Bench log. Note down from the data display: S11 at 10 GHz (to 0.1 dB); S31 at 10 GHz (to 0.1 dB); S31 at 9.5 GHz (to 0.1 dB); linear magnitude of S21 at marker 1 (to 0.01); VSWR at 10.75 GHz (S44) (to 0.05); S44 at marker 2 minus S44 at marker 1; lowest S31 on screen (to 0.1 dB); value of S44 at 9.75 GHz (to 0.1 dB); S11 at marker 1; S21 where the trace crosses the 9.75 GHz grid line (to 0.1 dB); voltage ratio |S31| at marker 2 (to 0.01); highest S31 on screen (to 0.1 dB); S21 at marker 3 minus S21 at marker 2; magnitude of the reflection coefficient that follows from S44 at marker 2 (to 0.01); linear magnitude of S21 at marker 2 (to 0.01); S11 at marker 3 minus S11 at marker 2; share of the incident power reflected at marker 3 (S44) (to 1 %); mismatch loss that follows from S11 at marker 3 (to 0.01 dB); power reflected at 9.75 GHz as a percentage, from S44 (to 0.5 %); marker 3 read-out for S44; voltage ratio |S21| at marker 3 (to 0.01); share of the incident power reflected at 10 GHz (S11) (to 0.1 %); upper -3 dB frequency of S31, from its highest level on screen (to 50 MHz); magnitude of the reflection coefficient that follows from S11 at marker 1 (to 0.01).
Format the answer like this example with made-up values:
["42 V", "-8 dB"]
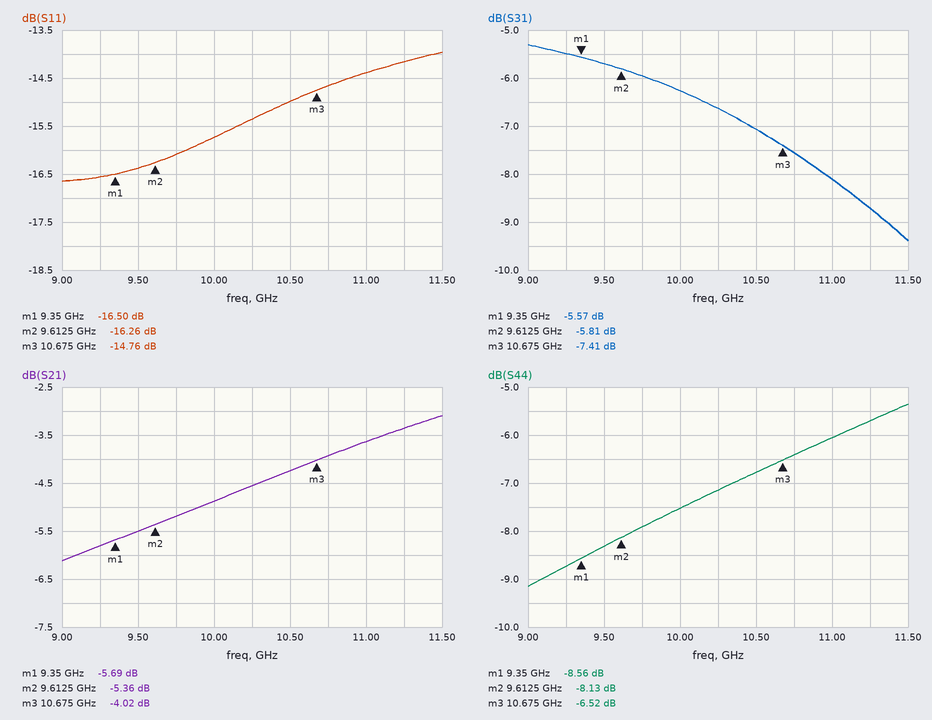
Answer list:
["-15.7 dB", "-6.3 dB", "-5.7 dB", "0.52", "2.85", "0.43 dB", "-9.4 dB", "-7.9 dB", "-16.50 dB", "-5.2 dB", "0.51", "-5.3 dB", "1.34 dB", "0.39", "0.54", "1.50 dB", "22 %", "0.15 dB", "16.0 %", "-6.52 dB", "0.63", "2.7 %", "11.10 GHz", "0.15"]
